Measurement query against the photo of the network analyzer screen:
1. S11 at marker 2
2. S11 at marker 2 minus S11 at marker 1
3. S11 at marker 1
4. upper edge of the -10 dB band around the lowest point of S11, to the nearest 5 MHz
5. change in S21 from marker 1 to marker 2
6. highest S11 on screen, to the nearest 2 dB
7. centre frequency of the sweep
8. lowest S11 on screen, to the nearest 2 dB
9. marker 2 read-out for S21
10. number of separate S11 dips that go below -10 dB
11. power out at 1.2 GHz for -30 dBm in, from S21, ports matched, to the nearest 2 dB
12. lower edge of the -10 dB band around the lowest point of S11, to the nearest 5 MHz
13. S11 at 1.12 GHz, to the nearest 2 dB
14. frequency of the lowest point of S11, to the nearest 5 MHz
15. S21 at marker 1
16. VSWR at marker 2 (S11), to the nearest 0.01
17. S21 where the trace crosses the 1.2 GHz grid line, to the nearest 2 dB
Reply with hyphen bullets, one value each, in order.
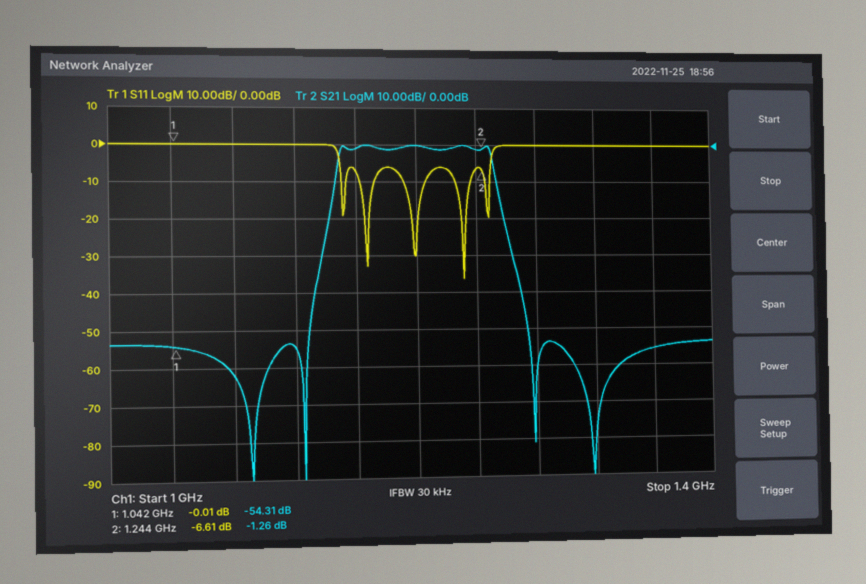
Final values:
- -6.61 dB
- -6.60 dB
- -0.01 dB
- 1.235 GHz
- 53.05 dB
- 0 dB
- 1.2 GHz
- -36 dB
- -1.26 dB
- 5
- -30 dBm
- 1.225 GHz
- 0 dB
- 1.230 GHz
- -54.31 dB
- 2.75
- 0 dB
